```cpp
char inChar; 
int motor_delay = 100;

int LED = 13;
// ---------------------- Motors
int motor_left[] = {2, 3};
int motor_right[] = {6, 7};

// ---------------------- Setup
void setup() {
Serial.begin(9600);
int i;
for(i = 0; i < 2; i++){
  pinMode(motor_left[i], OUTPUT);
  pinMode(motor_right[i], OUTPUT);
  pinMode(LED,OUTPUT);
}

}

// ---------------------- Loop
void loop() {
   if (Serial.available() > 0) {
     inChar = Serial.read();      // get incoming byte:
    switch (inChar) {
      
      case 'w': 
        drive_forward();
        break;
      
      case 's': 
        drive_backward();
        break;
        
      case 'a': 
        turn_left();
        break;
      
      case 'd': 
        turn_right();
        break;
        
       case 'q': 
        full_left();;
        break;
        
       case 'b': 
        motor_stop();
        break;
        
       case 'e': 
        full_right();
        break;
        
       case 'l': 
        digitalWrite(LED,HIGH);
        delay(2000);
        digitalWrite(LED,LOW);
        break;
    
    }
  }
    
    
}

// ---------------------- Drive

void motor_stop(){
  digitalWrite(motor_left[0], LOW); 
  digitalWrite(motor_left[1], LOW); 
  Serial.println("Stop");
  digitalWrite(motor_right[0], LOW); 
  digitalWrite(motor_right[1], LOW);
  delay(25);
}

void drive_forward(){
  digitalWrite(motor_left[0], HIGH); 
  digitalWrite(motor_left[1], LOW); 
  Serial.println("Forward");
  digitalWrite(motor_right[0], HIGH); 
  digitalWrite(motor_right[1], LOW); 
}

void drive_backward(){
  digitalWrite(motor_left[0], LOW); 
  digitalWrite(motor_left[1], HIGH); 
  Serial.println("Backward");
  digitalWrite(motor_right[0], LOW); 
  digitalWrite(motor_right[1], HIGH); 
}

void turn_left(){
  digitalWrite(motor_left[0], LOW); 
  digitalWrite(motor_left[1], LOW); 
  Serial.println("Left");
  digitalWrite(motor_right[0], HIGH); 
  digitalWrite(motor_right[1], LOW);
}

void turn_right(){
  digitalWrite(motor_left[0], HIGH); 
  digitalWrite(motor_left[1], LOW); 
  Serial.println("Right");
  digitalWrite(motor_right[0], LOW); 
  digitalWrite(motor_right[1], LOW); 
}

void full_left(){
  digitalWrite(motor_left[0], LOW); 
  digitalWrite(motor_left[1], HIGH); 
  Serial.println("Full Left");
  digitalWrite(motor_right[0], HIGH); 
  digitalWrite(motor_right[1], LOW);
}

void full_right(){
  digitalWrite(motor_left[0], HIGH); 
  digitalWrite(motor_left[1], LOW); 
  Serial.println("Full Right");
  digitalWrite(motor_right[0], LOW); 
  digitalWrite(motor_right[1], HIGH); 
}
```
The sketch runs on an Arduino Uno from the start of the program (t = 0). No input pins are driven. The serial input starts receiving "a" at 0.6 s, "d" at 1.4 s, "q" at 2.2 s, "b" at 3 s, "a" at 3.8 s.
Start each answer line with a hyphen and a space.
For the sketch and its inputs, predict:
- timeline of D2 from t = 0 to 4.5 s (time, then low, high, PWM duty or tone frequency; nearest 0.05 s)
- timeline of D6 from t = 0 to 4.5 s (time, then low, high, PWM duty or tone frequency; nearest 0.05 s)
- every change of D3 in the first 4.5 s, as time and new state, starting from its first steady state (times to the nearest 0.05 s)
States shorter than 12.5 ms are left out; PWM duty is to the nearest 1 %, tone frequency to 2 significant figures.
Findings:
- 0 s low; 1.4 s high; 2.2 s low
- 0 s low; 0.6 s high; 1.4 s low; 2.2 s high; 3 s low; 3.8 s high
- 0 s low; 2.2 s high; 3 s low
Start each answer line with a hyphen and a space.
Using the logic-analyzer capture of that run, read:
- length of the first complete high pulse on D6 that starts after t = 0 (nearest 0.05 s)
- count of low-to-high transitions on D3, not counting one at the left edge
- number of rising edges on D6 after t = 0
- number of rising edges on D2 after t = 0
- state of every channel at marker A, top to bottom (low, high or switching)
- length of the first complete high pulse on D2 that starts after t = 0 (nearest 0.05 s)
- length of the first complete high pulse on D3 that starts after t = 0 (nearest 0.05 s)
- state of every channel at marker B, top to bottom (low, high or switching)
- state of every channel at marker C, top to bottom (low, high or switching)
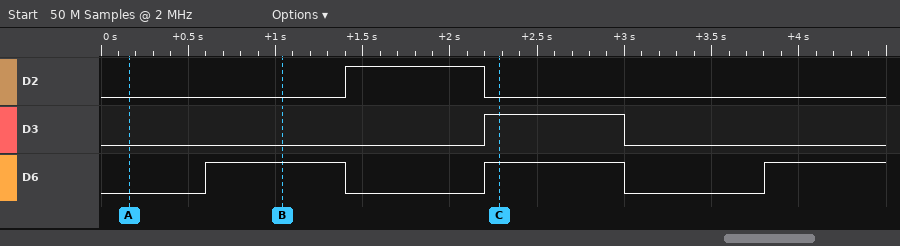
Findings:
- 0.80 s
- 1
- 3
- 1
- D2 low, D3 low, D6 low
- 0.80 s
- 0.80 s
- D2 low, D3 low, D6 high
- D2 low, D3 high, D6 high
